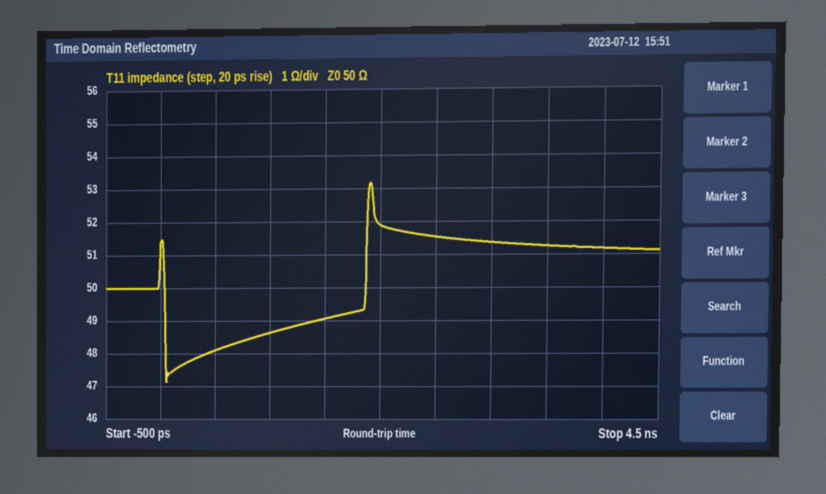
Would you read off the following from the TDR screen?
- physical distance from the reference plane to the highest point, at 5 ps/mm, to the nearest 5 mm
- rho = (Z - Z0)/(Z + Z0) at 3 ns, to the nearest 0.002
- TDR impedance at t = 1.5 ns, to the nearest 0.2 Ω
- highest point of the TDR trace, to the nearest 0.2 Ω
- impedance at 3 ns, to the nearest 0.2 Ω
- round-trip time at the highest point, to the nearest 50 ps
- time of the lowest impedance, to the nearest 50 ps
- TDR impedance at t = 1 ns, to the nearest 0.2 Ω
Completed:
190 mm
+0.014
49.0 Ω
53.2 Ω
51.4 Ω
1.90 ns
50 ps
48.6 Ω
